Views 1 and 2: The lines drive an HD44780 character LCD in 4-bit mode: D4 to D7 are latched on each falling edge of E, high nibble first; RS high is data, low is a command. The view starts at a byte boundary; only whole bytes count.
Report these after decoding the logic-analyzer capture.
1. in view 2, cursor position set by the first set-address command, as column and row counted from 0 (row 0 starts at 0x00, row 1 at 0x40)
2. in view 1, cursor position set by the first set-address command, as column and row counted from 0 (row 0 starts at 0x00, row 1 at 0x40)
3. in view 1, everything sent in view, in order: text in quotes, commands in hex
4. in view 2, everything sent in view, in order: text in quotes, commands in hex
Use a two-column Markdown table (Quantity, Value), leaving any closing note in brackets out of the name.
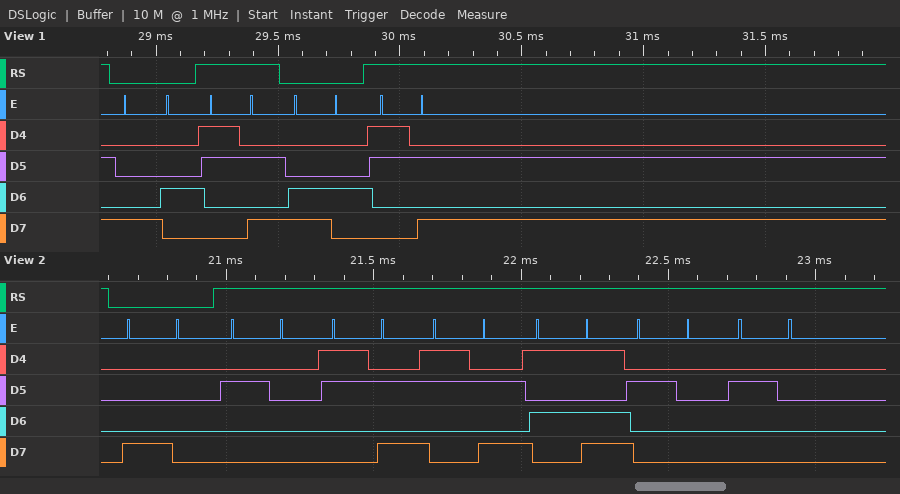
| Quantity | Value |
|---|---|
| in view 2, cursor position set by the first set-address command, as column and row counted from 0 | column 0, row 0 |
| in view 1, cursor position set by the first set-address command, as column and row counted from 0 | column 4, row 0 |
| in view 1, everything sent in view, in order: text in quotes, commands in hex | 0x84 ":" 0xC4 ":" |
| in view 2, everything sent in view, in order: text in quotes, commands in hex | 0x80 " ::]  " |
